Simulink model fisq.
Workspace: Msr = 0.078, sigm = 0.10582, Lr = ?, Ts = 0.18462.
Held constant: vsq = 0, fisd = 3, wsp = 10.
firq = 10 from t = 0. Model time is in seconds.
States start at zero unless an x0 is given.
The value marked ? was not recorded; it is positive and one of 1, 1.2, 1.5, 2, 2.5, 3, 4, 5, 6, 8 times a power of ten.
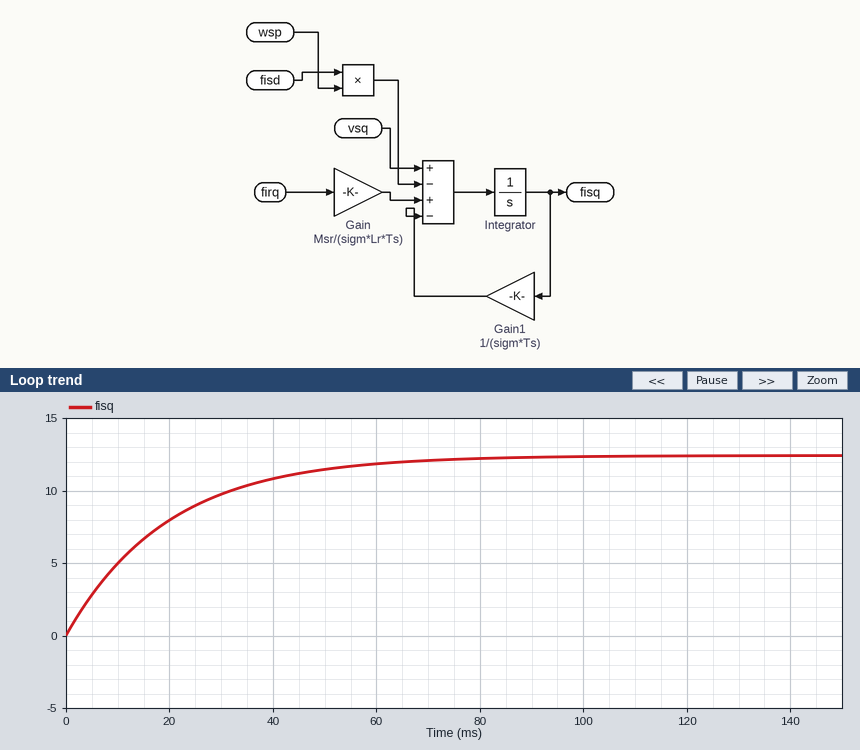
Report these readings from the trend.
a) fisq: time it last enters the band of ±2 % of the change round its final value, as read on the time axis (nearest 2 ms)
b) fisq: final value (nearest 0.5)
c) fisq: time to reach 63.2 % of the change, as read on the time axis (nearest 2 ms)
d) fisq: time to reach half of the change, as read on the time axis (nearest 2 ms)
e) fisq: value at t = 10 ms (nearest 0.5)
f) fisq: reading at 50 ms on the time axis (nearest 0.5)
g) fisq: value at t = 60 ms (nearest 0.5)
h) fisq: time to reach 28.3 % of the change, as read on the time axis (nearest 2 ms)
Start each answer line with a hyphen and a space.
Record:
- 76 ms
- 12.5
- 20 ms
- 14 ms
- 5.0
- 11.5
- 12.0
- 6 ms
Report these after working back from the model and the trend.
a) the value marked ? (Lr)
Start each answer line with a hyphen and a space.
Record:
- 0.06
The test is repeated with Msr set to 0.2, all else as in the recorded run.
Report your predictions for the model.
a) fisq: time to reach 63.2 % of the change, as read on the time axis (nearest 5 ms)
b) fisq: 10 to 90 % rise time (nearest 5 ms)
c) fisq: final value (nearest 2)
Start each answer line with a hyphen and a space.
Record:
- 20 ms
- 45 ms
- 32
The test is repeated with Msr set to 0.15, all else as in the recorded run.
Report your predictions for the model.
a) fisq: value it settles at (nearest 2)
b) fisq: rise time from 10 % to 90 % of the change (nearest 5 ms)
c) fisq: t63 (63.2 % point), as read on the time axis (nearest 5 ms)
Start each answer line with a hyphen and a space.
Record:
- 24
- 45 ms
- 20 ms
